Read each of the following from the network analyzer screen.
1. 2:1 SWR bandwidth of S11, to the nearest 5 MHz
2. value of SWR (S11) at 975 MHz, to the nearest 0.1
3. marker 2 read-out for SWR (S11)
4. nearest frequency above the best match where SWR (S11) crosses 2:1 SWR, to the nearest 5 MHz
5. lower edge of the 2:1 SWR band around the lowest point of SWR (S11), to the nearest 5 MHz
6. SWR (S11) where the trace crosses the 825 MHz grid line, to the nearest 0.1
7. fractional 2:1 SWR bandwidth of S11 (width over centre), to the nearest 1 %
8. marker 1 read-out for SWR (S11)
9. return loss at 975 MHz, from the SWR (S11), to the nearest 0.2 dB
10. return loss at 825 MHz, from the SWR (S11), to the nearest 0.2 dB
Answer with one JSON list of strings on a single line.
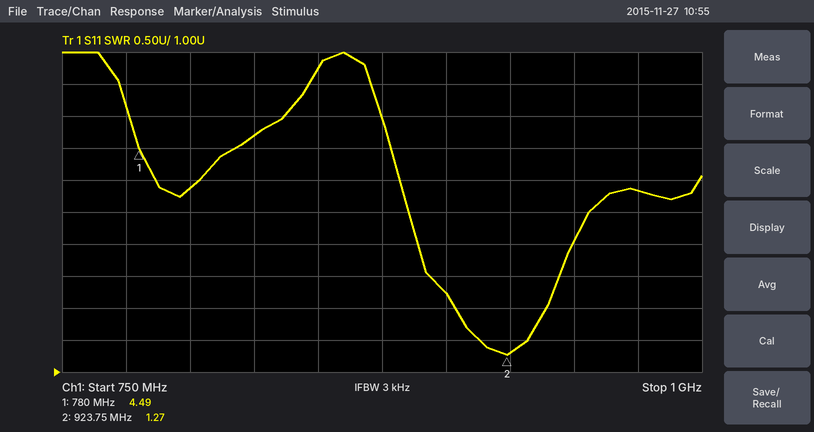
["35 MHz", "3.8", "1.27", "940 MHz", "905 MHz", "4.7", "4 %", "4.49", "4.6 dB", "3.8 dB"]
